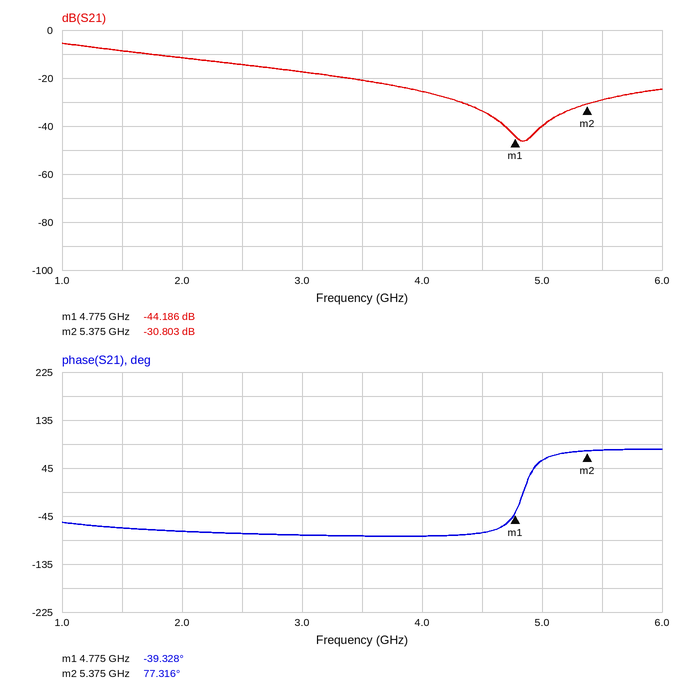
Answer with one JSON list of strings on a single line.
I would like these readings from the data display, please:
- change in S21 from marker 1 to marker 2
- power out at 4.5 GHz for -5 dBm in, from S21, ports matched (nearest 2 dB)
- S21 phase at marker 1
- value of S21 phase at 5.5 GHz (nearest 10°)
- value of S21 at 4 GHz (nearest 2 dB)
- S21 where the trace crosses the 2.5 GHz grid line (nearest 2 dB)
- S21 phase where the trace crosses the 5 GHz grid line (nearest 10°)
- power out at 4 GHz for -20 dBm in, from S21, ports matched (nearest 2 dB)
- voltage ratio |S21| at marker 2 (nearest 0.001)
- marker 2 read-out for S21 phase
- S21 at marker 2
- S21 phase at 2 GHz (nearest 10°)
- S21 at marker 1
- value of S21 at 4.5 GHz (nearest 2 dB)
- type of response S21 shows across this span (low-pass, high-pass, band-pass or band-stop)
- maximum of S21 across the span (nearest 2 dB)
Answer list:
["13.383 dB", "-38 dBm", "-39.328°", "80°", "-26 dB", "-14 dB", "60°", "-46 dBm", "0.029", "77.316°", "-30.803 dB", "-70°", "-44.186 dB", "-34 dB", "low-pass", "-6 dB"]
